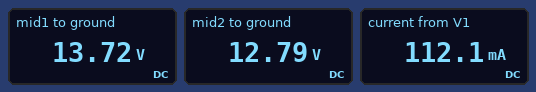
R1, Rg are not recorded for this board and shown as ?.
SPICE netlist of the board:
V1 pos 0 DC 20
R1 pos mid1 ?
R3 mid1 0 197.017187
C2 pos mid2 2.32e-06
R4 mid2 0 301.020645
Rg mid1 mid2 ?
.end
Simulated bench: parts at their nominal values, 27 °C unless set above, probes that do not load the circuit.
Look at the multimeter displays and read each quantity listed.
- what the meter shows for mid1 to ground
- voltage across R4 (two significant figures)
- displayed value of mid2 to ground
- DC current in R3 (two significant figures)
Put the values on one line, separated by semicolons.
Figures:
13.72 V; 13 V; 12.79 V; 70 mA
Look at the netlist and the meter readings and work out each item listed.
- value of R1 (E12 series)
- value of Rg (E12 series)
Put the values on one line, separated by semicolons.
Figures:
56 Ω; 22 Ω
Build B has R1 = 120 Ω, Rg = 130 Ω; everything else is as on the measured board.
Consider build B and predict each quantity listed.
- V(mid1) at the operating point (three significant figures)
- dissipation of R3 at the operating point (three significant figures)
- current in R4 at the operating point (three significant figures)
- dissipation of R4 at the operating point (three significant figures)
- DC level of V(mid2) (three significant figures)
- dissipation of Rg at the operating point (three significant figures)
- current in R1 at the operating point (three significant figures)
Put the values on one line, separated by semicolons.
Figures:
10.6 V; 570 mW; 24.6 mA; 182 mW; 7.40 V; 78.6 mW; 78.4 mA
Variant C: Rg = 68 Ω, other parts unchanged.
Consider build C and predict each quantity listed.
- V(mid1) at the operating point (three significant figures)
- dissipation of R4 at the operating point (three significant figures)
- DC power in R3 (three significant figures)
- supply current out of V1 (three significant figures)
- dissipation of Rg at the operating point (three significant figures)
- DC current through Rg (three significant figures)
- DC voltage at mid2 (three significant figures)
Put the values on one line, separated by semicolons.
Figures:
13.9 V; 429 mW; 985 mW; 108 mA; 96.9 mW; 37.7 mA; 11.4 V
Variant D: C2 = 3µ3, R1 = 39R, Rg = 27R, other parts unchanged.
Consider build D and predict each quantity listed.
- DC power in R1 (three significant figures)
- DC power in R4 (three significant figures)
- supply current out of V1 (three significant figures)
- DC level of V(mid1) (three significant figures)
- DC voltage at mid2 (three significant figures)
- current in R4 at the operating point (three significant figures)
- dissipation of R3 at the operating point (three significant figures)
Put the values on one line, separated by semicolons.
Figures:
594 mW; 645 mW; 123 mA; 15.2 V; 13.9 V; 46.3 mA; 1.17 W
